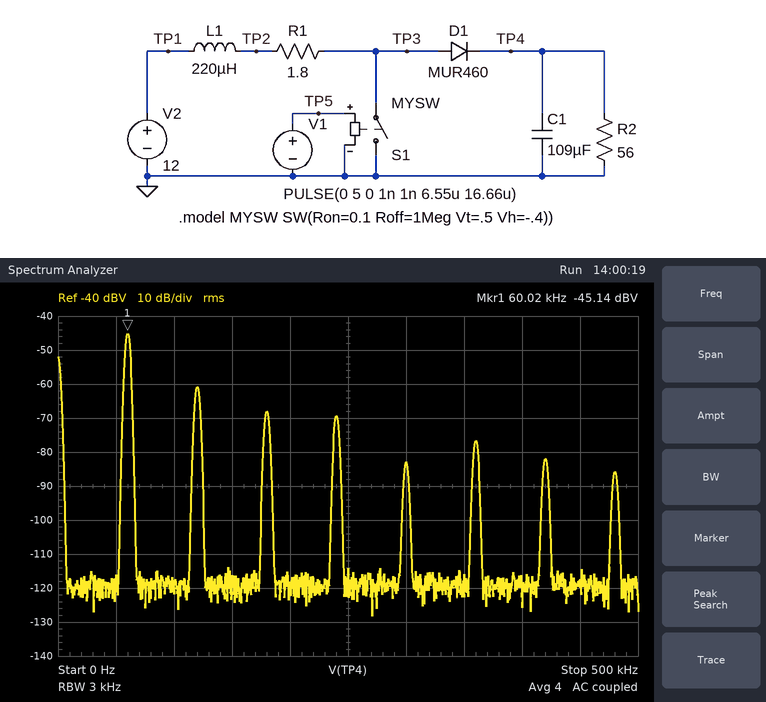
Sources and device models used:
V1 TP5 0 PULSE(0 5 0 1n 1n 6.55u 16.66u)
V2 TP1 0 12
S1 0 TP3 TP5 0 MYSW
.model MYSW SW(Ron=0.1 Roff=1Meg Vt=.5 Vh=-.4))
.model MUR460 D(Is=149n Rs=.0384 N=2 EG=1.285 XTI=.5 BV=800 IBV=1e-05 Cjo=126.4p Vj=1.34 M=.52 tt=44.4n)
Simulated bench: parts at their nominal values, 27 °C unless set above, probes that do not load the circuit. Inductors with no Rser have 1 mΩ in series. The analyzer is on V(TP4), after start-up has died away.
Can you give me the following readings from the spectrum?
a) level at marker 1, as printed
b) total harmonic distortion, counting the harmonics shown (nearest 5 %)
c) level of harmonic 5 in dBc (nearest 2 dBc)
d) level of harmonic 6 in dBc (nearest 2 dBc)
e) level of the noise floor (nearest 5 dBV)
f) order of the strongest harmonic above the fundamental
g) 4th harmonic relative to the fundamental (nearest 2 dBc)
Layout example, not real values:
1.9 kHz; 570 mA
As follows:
-45.14 dBV; 20 %; -38 dBc; -32 dBc; -120 dBV; 2; -24 dBc
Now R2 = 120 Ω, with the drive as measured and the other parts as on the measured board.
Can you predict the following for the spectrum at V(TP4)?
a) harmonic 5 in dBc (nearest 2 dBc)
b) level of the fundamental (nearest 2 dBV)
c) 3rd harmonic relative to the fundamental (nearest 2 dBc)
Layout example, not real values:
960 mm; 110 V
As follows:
-32 dBc; -50 dBV; -22 dBc
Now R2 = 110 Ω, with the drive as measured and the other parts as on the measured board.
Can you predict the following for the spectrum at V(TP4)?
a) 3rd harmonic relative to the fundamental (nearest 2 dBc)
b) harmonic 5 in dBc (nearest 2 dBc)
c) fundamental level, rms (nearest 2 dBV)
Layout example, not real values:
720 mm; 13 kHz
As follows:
-22 dBc; -32 dBc; -50 dBV
